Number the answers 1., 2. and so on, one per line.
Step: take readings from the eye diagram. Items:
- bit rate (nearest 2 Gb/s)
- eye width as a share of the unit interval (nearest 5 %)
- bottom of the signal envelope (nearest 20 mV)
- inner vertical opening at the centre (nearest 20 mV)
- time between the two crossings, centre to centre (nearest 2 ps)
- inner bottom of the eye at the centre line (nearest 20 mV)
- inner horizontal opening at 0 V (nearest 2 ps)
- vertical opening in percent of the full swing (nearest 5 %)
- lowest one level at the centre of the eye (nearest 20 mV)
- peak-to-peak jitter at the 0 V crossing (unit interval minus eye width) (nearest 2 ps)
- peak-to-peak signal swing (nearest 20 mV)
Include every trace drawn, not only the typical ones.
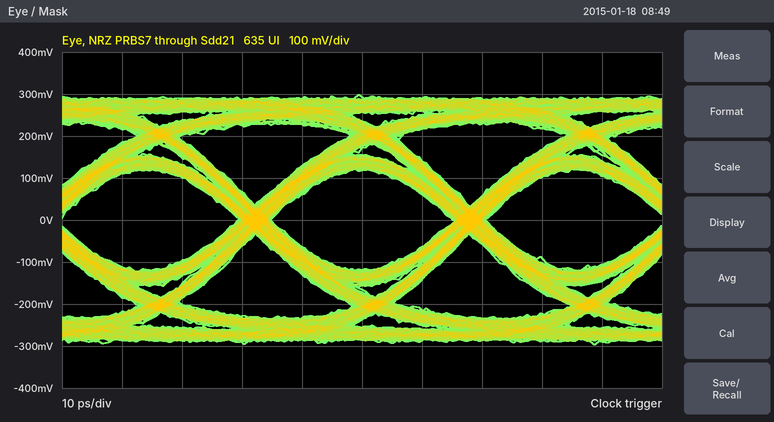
1. 28 Gb/s
2. 85 %
3. -300 mV
4. 240 mV
5. 36 ps
6. -120 mV
7. 30 ps
8. 40 %
9. 120 mV
10. 6 ps
11. 600 mV
